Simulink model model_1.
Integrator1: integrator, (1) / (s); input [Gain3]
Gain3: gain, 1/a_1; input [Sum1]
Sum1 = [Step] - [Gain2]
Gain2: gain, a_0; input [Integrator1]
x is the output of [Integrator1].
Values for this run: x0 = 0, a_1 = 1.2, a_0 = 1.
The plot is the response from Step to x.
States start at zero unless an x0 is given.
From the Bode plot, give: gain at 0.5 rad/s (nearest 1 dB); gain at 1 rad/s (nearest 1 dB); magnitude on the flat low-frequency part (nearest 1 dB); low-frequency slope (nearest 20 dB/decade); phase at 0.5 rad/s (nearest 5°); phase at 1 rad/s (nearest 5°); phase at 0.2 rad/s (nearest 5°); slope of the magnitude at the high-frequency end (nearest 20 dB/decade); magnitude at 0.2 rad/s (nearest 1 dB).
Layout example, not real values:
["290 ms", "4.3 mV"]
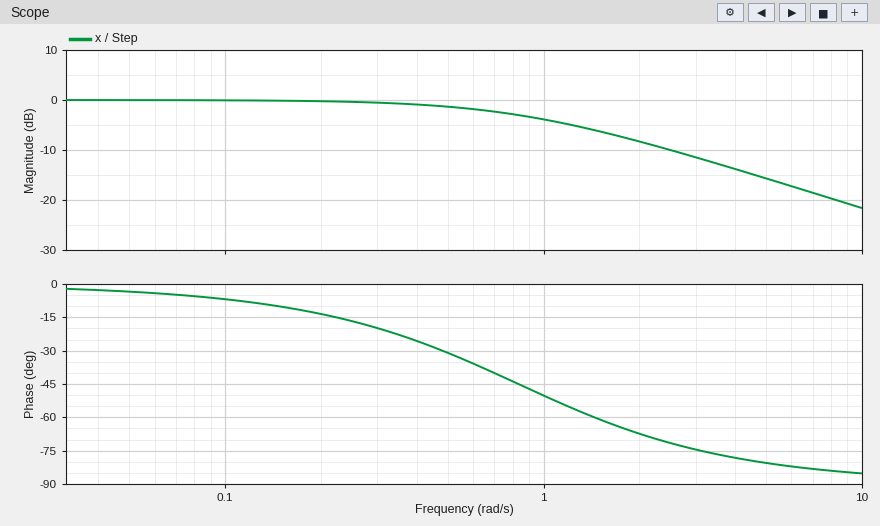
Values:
["-1 dB", "-4 dB", "0 dB", "0 dB/decade", "-30°", "-50°", "-15°", "-20 dB/decade", "0 dB"]
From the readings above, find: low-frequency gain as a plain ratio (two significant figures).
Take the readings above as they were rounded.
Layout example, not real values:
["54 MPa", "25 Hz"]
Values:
["1.0"]
